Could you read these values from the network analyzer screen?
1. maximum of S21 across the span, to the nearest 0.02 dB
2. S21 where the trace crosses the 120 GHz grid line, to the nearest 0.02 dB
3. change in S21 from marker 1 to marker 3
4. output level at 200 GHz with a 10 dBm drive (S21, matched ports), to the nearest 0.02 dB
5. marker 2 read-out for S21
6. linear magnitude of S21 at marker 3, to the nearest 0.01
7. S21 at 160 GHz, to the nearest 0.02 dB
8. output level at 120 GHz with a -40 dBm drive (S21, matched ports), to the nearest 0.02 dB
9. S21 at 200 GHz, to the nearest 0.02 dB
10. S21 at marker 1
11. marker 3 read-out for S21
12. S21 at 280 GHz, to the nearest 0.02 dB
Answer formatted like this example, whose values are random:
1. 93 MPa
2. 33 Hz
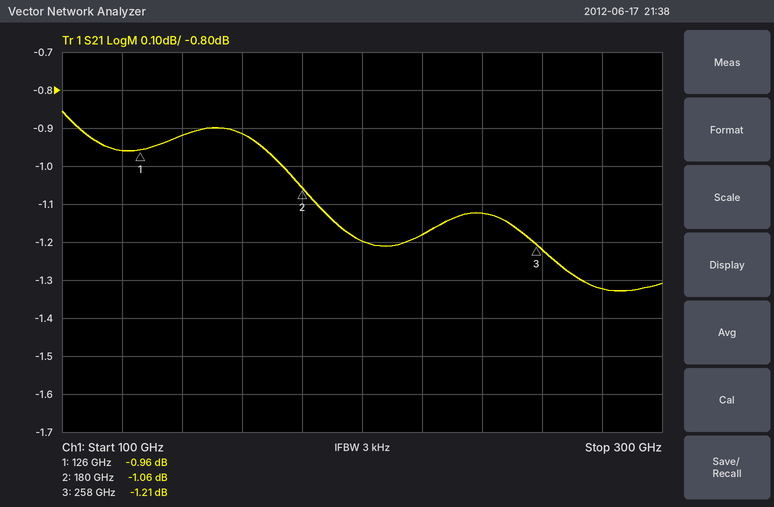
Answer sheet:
1. -0.86 dB
2. -0.96 dB
3. -0.25 dB
4. 8.80 dBm
5. -1.06 dB
6. 0.87
7. -0.92 dB
8. -40.96 dBm
9. -1.20 dB
10. -0.96 dB
11. -1.21 dB
12. -1.32 dB
